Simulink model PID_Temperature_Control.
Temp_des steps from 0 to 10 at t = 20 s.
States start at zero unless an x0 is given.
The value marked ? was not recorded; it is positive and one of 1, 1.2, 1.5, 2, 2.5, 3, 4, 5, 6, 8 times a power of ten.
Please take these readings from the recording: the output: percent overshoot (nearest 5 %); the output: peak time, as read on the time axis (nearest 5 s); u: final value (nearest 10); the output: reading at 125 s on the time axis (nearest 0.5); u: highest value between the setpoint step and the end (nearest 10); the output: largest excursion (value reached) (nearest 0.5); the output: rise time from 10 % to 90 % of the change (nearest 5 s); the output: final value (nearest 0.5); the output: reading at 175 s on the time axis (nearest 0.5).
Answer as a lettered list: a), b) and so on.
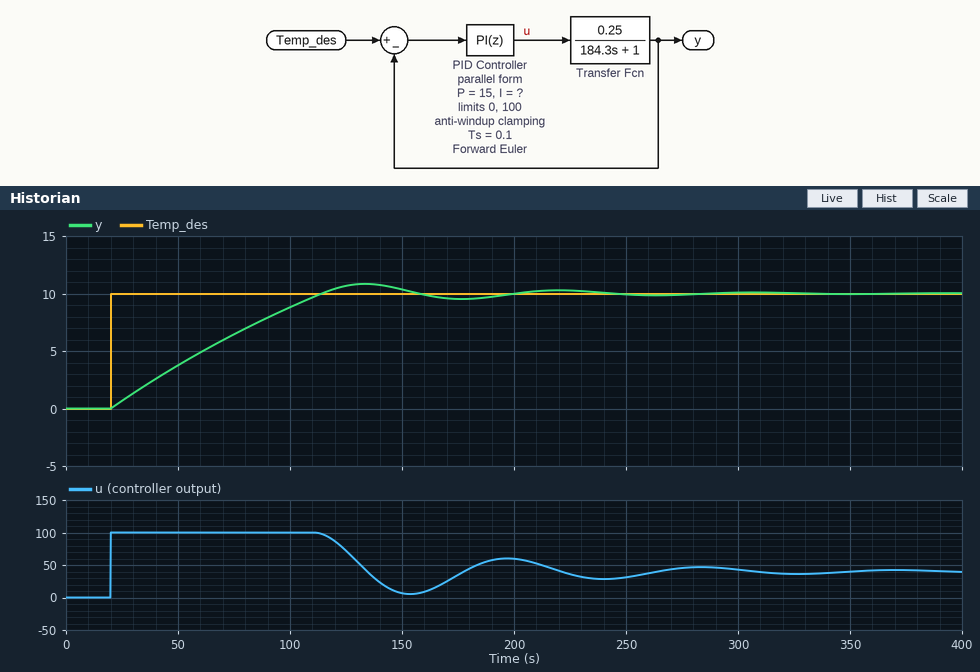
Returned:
a) 10 %
b) 135 s
c) 40
d) 10.5
e) 100
f) 11.0
g) 75 s
h) 10.0
i) 9.5
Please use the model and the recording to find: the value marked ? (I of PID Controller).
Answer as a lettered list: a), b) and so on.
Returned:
a) 4
